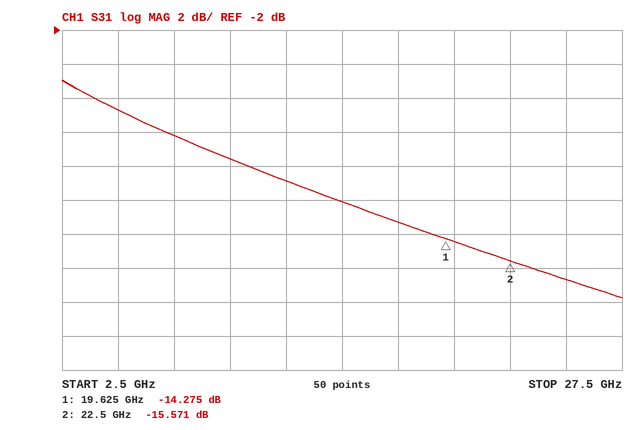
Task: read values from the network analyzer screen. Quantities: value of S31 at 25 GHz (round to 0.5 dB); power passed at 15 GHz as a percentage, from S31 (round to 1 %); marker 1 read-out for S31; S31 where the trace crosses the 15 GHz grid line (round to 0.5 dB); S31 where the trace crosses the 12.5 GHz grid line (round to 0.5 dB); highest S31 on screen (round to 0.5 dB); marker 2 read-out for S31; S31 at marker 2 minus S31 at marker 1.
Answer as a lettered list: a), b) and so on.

a) -16.5 dB
b) 6 %
c) -14.275 dB
d) -12.0 dB
e) -11.0 dB
f) -5.0 dB
g) -15.571 dB
h) -1.296 dB
